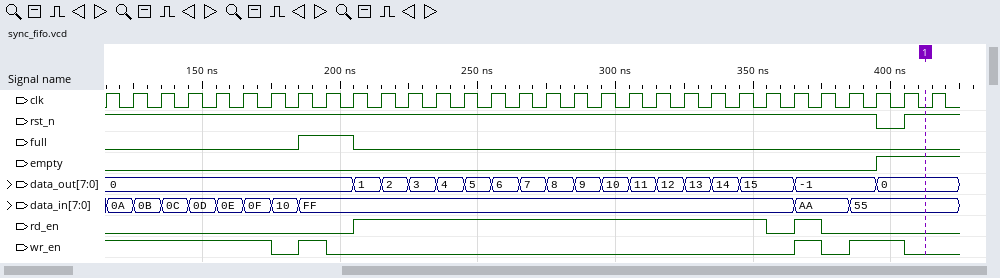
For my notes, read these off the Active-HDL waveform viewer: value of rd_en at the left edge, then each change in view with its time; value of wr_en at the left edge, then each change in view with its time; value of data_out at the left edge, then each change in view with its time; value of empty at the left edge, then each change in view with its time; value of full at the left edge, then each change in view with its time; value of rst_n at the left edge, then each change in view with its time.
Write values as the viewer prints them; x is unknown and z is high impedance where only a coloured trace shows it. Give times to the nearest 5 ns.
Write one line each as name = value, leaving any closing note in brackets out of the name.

value of rd_en at the left edge, then each change in view with its time = 0, 1 at 205 ns, 0 at 355 ns, 1 at 365 ns, 0 at 375 ns
value of wr_en at the left edge, then each change in view with its time = 1, 0 at 175 ns, 1 at 185 ns, 0 at 195 ns, 1 at 365 ns, 0 at 375 ns, 1 at 385 ns, 0 at 405 ns
value of data_out at the left edge, then each change in view with its time = 0, 1 at 205 ns, 2 at 215 ns, 3 at 225 ns, 4 at 235 ns, 5 at 245 ns, 6 at 255 ns, 7 at 265 ns, 8 at 275 ns, 9 at 285 ns, 10 at 295 ns, 11 at 305 ns, 12 at 315 ns, 13 at 325 ns, 14 at 335 ns, 15 at 345 ns, -1 at 365 ns, 0 at 395 ns
value of empty at the left edge, then each change in view with its time = 0, 1 at 395 ns
value of full at the left edge, then each change in view with its time = 0, 1 at 185 ns, 0 at 205 ns
value of rst_n at the left edge, then each change in view with its time = 1, 0 at 395 ns, 1 at 405 ns
